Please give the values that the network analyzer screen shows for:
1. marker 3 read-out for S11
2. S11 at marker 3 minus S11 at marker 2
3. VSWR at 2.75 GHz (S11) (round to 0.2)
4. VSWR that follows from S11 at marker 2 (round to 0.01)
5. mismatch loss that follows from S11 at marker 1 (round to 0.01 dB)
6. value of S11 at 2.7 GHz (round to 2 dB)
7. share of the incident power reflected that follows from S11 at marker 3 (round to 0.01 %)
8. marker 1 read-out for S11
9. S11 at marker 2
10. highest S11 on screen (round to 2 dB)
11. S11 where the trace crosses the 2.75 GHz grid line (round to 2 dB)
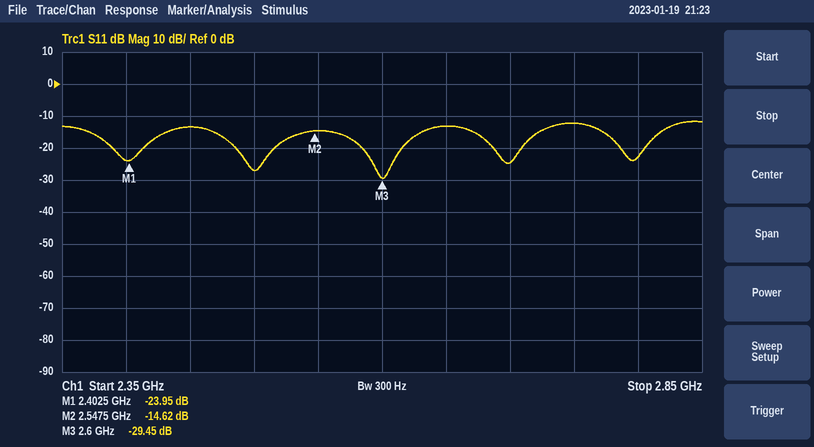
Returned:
-29.45 dB
-14.83 dB
1.6
1.46
0.02 dB
-24 dB
0.11 %
-23.95 dB
-14.62 dB
-12 dB
-12 dB
